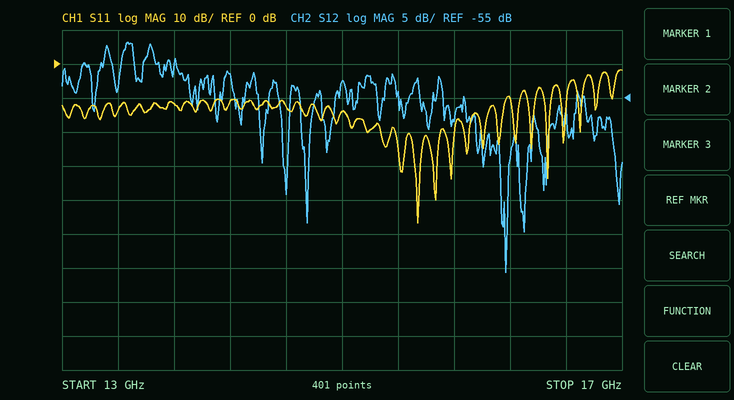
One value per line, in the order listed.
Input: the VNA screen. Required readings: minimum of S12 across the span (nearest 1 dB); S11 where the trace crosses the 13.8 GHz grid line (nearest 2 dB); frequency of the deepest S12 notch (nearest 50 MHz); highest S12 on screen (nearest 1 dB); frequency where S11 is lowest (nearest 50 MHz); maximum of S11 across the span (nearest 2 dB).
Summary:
-81 dB
-12 dB
16.15 GHz
-47 dB
15.55 GHz
-2 dB
